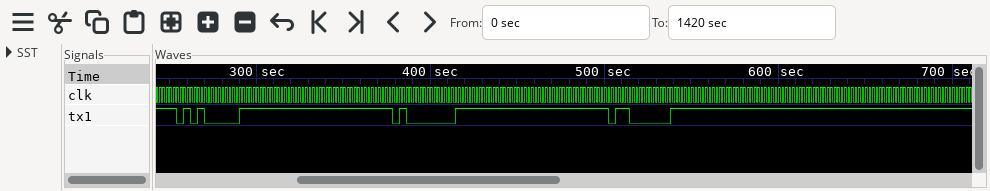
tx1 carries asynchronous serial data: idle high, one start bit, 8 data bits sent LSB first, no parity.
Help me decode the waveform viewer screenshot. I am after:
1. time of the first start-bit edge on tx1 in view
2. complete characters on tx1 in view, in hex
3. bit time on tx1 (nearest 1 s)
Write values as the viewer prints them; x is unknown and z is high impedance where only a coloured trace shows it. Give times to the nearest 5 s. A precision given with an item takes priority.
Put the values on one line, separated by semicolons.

255 s; 05, 01, 03; 4 s
